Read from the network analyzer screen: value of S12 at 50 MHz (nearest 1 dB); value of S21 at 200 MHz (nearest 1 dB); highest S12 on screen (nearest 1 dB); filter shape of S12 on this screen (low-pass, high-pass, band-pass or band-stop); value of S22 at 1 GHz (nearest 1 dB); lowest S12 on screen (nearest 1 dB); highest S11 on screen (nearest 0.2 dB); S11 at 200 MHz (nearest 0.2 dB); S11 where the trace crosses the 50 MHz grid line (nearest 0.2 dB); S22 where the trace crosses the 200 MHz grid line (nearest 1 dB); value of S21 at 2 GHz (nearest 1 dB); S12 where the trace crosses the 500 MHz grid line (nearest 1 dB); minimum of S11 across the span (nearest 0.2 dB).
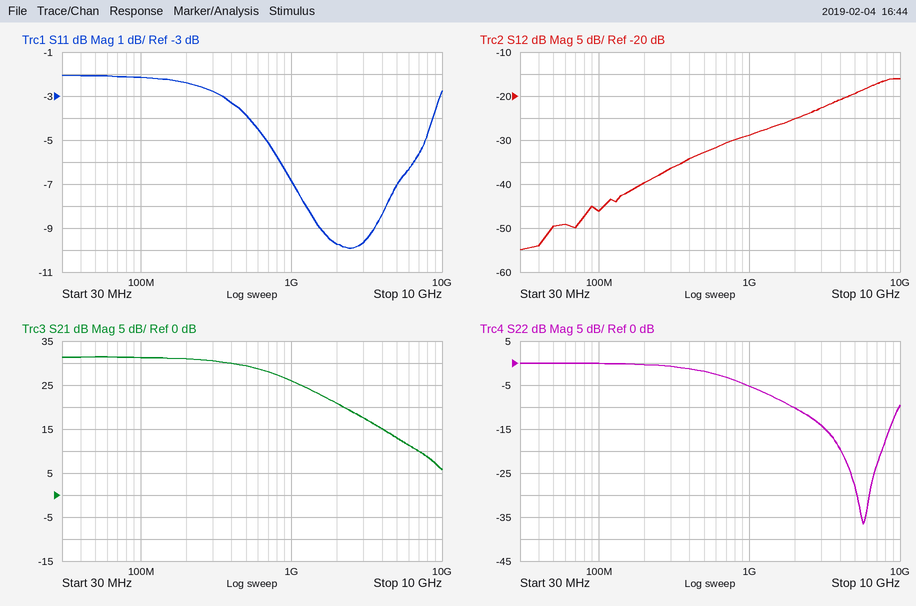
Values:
-50 dB
31 dB
-16 dB
high-pass
-5 dB
-55 dB
-2.0 dB
-2.4 dB
-2.0 dB
0 dB
21 dB
-33 dB
-10.0 dB
